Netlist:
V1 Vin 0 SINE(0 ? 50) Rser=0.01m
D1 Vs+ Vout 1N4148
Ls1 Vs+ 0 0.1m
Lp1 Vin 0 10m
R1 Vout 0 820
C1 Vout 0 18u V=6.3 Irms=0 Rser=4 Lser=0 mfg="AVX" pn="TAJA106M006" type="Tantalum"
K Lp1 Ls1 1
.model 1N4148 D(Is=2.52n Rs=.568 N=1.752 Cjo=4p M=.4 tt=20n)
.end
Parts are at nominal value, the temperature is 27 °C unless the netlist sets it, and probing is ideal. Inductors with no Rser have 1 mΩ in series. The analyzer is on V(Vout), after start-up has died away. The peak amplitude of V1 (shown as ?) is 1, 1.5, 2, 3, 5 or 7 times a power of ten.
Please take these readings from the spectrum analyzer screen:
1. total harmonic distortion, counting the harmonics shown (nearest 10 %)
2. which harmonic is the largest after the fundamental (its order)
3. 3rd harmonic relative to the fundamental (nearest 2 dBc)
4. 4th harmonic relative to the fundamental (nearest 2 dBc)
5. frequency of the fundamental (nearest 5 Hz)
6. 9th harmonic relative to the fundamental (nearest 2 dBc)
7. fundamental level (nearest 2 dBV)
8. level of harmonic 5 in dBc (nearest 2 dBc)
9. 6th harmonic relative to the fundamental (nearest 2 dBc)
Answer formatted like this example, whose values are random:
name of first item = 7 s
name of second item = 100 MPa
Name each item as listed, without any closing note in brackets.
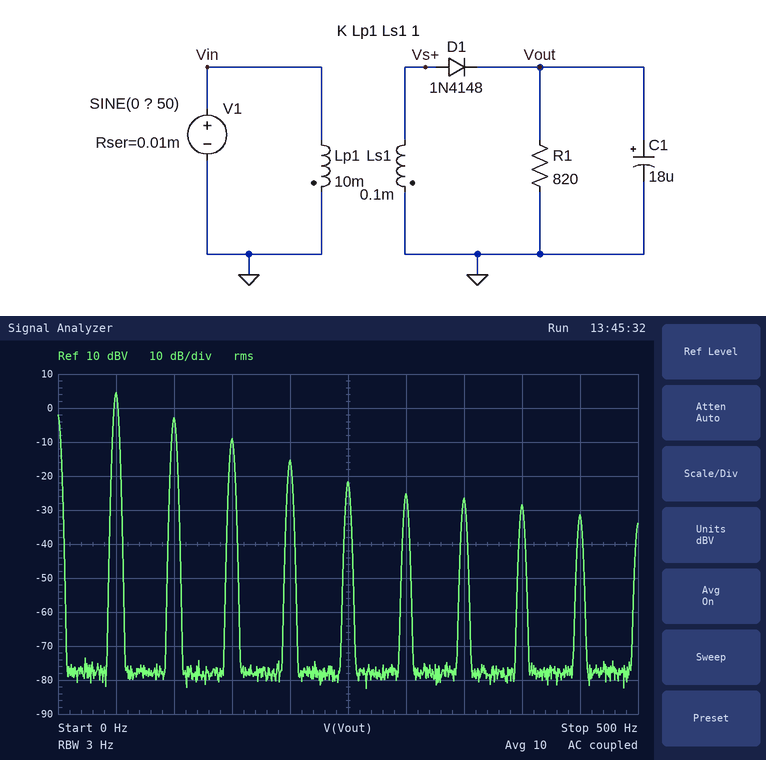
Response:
total harmonic distortion, counting the harmonics shown = 50 %
which harmonic is the largest after the fundamental = 2
3rd harmonic relative to the fundamental = -14 dBc
4th harmonic relative to the fundamental = -20 dBc
frequency of the fundamental = 50 Hz
9th harmonic relative to the fundamental = -36 dBc
fundamental level = 4 dBV
level of harmonic 5 in dBc = -26 dBc
6th harmonic relative to the fundamental = -30 dBc
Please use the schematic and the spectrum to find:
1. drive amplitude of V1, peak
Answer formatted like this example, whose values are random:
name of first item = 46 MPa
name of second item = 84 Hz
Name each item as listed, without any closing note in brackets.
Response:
drive amplitude of V1, peak = 100 V
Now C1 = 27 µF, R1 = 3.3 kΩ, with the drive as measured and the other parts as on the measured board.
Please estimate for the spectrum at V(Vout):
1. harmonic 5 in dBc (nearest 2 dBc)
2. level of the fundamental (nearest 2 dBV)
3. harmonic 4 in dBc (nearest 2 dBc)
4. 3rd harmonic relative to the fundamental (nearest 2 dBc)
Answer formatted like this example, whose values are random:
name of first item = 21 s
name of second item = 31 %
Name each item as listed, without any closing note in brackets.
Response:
harmonic 5 in dBc = -16 dBc
level of the fundamental = -8 dBV
harmonic 4 in dBc = -14 dBc
3rd harmonic relative to the fundamental = -10 dBc
